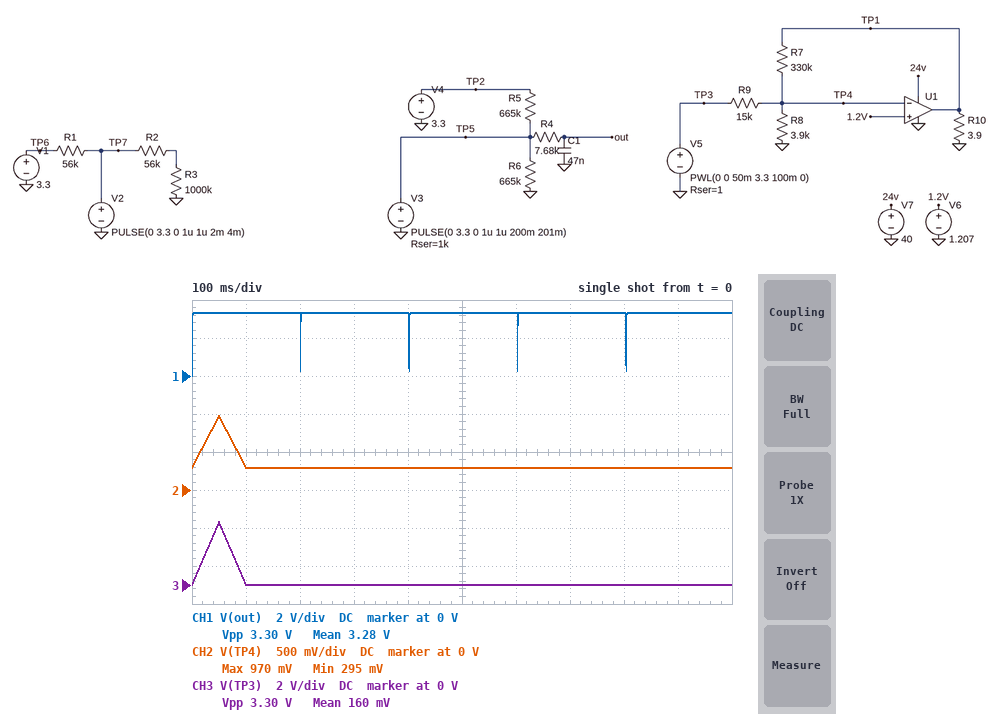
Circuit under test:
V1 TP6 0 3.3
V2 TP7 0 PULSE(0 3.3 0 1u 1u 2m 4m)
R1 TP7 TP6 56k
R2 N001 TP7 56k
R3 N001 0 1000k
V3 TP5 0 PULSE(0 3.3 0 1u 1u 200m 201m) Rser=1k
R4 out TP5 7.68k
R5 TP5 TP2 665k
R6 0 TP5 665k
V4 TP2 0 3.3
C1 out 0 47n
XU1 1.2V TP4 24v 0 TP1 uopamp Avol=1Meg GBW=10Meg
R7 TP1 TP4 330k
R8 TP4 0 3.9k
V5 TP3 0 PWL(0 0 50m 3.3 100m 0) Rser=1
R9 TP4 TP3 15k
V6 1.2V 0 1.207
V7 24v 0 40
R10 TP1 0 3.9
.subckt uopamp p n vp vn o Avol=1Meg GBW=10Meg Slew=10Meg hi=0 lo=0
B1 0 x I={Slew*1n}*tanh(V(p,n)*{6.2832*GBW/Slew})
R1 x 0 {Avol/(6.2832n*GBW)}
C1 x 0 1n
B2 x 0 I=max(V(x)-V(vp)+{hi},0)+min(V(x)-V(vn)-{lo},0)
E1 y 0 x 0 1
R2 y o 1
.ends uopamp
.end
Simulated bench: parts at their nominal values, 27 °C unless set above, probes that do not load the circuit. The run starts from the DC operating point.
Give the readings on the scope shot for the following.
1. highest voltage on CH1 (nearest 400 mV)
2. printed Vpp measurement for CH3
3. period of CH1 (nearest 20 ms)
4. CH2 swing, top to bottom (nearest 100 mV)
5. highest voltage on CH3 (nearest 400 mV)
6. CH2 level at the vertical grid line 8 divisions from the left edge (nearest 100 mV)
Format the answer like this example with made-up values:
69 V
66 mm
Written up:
3.2 V
3.30 V
200 ms
700 mV
3.2 V
300 mV
